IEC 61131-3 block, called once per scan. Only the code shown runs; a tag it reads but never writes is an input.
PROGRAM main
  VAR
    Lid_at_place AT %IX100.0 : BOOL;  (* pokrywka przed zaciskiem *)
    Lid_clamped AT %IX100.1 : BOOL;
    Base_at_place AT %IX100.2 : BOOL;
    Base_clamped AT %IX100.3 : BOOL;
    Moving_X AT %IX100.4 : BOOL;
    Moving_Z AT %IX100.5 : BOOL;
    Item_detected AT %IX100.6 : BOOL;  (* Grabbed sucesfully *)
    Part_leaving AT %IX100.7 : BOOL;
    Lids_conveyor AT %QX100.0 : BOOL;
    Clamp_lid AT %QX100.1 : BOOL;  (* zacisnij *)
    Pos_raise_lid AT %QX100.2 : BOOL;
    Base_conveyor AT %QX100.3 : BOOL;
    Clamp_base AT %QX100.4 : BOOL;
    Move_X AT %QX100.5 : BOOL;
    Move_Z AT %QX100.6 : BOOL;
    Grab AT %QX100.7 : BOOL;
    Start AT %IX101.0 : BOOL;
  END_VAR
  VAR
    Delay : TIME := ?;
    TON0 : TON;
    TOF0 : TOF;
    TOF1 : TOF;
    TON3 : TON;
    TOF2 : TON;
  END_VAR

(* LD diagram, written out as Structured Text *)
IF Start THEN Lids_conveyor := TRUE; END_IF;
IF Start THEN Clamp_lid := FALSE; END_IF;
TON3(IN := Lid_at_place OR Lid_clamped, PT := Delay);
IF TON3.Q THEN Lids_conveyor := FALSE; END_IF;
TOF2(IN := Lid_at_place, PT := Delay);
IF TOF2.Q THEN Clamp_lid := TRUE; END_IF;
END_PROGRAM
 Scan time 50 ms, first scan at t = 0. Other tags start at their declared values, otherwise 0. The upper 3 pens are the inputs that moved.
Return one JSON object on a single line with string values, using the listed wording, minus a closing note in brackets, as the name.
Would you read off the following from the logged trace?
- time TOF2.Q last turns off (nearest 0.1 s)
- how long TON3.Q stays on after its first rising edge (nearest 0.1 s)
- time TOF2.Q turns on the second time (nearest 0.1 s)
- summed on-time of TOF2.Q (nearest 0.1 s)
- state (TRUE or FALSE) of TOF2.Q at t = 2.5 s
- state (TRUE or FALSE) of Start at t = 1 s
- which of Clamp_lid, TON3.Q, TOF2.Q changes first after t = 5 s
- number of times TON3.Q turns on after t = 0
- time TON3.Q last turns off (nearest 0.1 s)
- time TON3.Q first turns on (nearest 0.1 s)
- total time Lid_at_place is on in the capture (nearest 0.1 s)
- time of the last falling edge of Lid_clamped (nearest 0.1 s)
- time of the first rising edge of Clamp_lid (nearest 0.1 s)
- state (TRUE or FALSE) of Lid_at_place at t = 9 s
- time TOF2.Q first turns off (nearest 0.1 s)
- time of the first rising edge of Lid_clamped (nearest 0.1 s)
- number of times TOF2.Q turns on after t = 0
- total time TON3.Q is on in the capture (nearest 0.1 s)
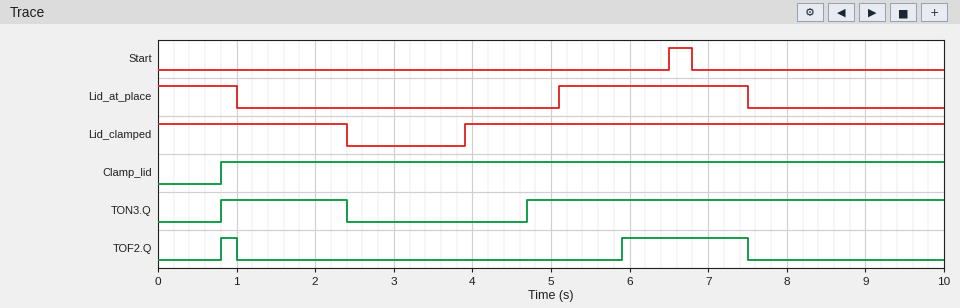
{"time TOF2.Q last turns off": "7.5 s", "how long TON3.Q stays on after its first rising edge": "1.6 s", "time TOF2.Q turns on the second time": "5.9 s", "summed on-time of TOF2.Q": "1.8 s", "state (TRUE or FALSE) of TOF2.Q at t = 2.5 s": "FALSE", "state (TRUE or FALSE) of Start at t = 1 s": "FALSE", "which of Clamp_lid, TON3.Q, TOF2.Q changes first after t = 5 s": "TOF2.Q", "number of times TON3.Q turns on after t = 0": "2", "time TON3.Q last turns off": "2.4 s", "time TON3.Q first turns on": "0.8 s", "total time Lid_at_place is on in the capture": "3.4 s", "time of the last falling edge of Lid_clamped": "2.4 s", "time of the first rising edge of Clamp_lid": "0.8 s", "state (TRUE or FALSE) of Lid_at_place at t = 9 s": "FALSE", "time TOF2.Q first turns off": "1.0 s", "time of the first rising edge of Lid_clamped": "3.9 s", "number of times TOF2.Q turns on after t = 0": "2", "total time TON3.Q is on in the capture": "6.9 s"}
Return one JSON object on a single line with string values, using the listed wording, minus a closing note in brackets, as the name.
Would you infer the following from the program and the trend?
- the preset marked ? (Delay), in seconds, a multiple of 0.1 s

{"the preset marked ? (Delay), in seconds, a multiple of 0.1 s": "0.8 s"}
